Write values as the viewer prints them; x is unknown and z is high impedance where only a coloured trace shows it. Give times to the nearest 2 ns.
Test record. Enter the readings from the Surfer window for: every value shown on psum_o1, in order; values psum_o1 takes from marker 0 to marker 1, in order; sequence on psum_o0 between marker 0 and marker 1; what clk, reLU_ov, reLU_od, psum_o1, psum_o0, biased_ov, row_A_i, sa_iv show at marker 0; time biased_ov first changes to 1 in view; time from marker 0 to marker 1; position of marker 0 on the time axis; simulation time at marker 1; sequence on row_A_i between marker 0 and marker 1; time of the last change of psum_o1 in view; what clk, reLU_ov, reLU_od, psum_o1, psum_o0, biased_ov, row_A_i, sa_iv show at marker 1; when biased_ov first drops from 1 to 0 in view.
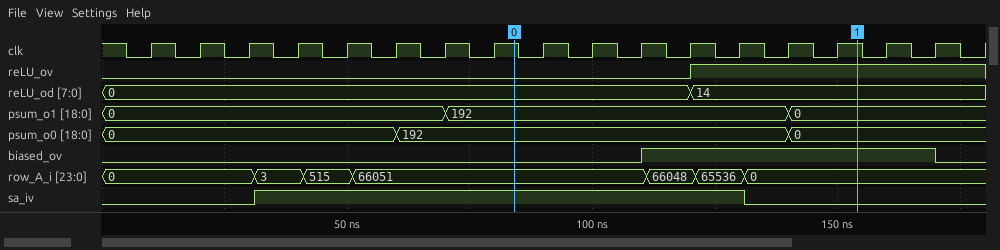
0, 192, 0
192, 0
192, 0
clk=1, reLU_ov=0, reLU_od=0, psum_o1=192, psum_o0=192, biased_ov=0, row_A_i=66051, sa_iv=1
110 ns
70 ns
84 ns
154 ns
66051, 66048, 65536, 0
140 ns
clk=1, reLU_ov=1, reLU_od=14, psum_o1=0, psum_o0=0, biased_ov=1, row_A_i=0, sa_iv=0
170 ns
